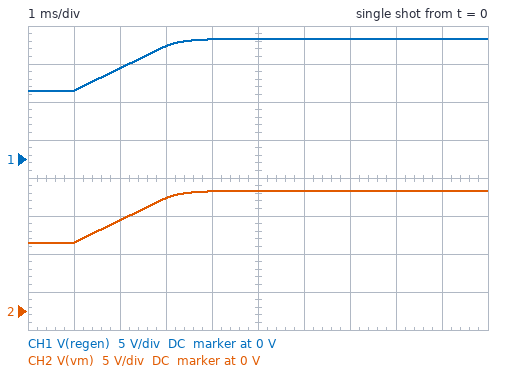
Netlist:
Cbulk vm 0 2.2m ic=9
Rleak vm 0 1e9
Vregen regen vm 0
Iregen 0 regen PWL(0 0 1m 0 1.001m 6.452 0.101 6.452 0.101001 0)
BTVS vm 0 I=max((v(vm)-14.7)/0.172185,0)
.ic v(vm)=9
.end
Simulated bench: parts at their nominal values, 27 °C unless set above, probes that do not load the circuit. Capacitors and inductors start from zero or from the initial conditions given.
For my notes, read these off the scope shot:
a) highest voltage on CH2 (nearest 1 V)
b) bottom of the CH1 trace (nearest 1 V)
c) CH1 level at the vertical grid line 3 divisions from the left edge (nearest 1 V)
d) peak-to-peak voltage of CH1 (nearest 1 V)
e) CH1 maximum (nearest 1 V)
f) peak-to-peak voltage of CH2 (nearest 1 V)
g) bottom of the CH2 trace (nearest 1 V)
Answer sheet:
16 V
9 V
15 V
7 V
16 V
7 V
9 V
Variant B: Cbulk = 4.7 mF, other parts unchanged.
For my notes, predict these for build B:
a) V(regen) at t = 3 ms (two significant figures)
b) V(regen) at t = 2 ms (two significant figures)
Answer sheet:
12 V
10 V
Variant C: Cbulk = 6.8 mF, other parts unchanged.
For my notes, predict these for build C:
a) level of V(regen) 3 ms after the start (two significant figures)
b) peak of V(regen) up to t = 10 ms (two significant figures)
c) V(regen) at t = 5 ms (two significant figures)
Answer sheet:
11 V
16 V
13 V
